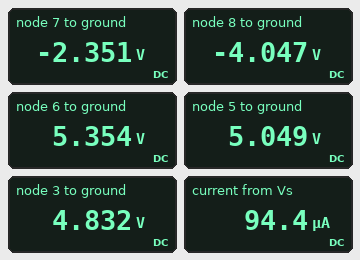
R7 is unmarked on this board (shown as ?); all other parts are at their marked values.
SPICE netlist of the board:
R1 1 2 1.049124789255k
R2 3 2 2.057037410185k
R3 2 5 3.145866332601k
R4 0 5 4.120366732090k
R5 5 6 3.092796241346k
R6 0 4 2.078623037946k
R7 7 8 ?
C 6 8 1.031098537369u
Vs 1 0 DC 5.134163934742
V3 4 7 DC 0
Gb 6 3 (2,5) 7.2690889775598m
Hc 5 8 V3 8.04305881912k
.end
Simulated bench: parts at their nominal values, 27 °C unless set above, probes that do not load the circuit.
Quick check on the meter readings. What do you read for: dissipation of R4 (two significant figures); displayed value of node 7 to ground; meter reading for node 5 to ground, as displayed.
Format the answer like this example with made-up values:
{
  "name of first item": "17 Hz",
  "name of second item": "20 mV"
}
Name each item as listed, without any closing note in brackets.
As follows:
{
  "dissipation of R4": "6.2 mW",
  "displayed value of node 7 to ground": "-2.351 V",
  "meter reading for node 5 to ground, as displayed": "5.049 V"
}
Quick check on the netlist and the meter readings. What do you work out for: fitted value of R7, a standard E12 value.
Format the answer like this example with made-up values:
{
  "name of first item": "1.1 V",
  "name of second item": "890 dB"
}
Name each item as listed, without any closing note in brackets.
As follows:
{
  "fitted value of R7, a standard E12 value": "1.5 kΩ"
}
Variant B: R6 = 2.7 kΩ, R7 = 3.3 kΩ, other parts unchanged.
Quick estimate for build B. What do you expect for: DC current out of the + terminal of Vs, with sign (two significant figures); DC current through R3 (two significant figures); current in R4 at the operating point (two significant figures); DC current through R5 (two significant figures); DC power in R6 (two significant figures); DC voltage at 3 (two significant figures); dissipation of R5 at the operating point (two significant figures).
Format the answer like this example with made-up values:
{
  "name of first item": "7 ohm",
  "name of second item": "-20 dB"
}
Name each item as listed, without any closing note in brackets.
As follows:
{
  "DC current out of the + terminal of Vs, with sign": "-1.6 mA",
  "DC current through R3": "75 µA",
  "current in R4 at the operating point": "1.6 mA",
  "DC current through R5": "1.7 mA",
  "DC power in R6": "28 mW",
  "DC voltage at 3": "10 V",
  "dissipation of R5 at the operating point": "9.0 mW"
}
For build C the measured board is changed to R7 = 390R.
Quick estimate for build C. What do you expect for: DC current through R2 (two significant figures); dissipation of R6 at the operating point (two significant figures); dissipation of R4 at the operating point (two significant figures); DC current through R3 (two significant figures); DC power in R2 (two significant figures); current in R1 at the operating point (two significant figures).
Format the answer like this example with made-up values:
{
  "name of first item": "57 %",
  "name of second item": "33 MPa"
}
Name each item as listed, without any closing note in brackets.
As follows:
{
  "DC current through R2": "320 µA",
  "dissipation of R6 at the operating point": "1.6 mW",
  "dissipation of R4 at the operating point": "5.7 mW",
  "DC current through R3": "14 µA",
  "DC power in R2": "210 µW",
  "current in R1 at the operating point": "310 µA"
}
